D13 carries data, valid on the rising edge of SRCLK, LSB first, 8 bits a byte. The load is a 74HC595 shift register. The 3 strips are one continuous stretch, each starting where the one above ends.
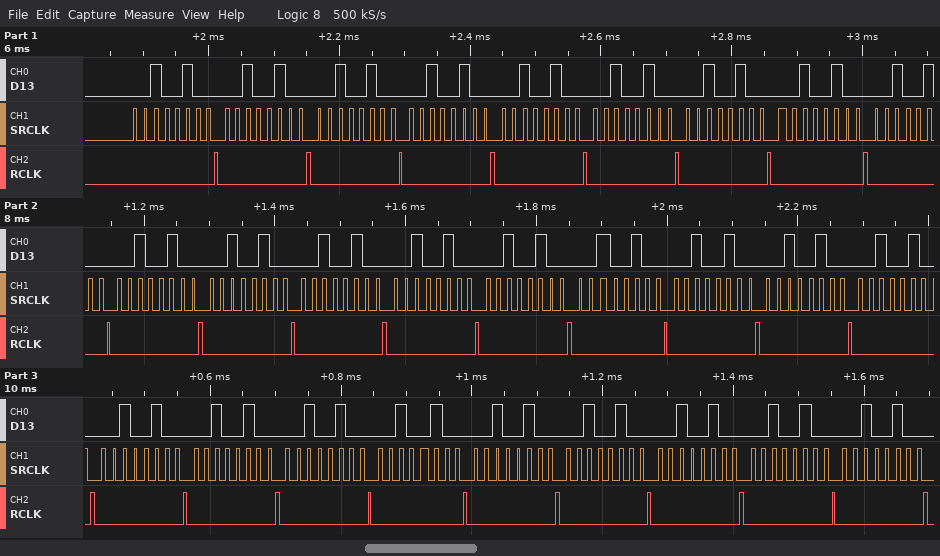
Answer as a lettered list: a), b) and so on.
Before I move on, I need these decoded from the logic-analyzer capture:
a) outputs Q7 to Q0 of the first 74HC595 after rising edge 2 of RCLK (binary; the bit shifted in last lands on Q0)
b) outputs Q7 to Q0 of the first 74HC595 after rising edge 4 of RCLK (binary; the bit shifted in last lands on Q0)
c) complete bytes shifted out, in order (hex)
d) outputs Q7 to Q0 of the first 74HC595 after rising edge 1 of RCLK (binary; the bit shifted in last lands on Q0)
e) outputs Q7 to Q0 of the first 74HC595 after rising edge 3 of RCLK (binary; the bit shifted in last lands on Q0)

a) 00100100
b) 00100100
c) 24 24 24 24 24 24 24 24 24 24 24 24 24 24 24 24 24 24 24 24 24 24 24 24 24 24 24
d) 00100100
e) 00100100
